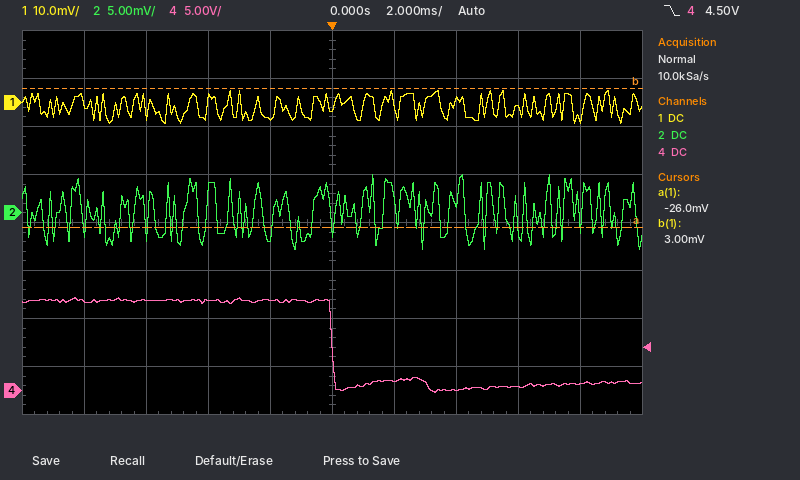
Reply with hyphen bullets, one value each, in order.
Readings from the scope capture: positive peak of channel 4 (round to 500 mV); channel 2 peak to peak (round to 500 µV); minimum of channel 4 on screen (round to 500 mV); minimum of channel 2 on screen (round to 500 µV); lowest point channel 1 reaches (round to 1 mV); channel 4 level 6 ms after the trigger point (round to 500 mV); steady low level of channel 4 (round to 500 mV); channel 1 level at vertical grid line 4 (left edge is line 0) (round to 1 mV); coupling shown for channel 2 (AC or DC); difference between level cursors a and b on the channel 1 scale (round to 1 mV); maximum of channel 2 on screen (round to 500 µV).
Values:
- 9.5 V
- 8.0 mV
- 0.0 V
- -4.0 mV
- -4 mV
- 500 mV
- 500 mV
- -3 mV
- DC
- 29 mV
- 4.0 mV
